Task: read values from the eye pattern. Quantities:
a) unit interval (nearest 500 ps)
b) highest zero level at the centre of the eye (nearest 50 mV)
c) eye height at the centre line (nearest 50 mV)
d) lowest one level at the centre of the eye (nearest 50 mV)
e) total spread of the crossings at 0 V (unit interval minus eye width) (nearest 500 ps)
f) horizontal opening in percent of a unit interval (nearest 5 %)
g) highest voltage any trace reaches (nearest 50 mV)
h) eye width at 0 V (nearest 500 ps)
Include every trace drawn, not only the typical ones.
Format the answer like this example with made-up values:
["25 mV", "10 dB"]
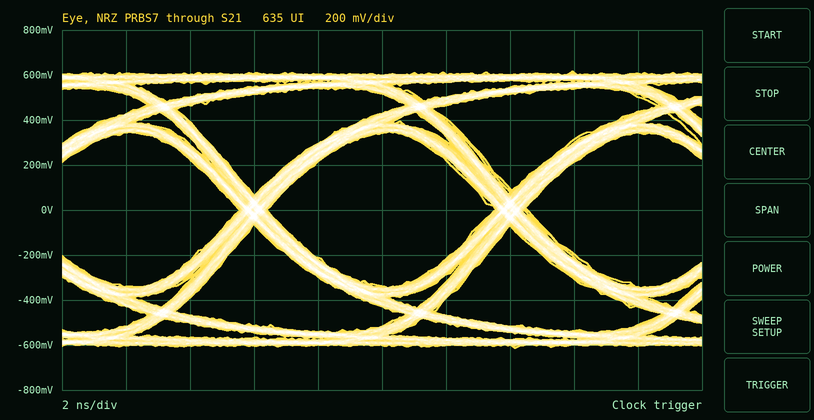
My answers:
["8.0 ns", "-350 mV", "700 mV", "350 mV", "1.0 ns", "90 %", "600 mV", "7.0 ns"]
